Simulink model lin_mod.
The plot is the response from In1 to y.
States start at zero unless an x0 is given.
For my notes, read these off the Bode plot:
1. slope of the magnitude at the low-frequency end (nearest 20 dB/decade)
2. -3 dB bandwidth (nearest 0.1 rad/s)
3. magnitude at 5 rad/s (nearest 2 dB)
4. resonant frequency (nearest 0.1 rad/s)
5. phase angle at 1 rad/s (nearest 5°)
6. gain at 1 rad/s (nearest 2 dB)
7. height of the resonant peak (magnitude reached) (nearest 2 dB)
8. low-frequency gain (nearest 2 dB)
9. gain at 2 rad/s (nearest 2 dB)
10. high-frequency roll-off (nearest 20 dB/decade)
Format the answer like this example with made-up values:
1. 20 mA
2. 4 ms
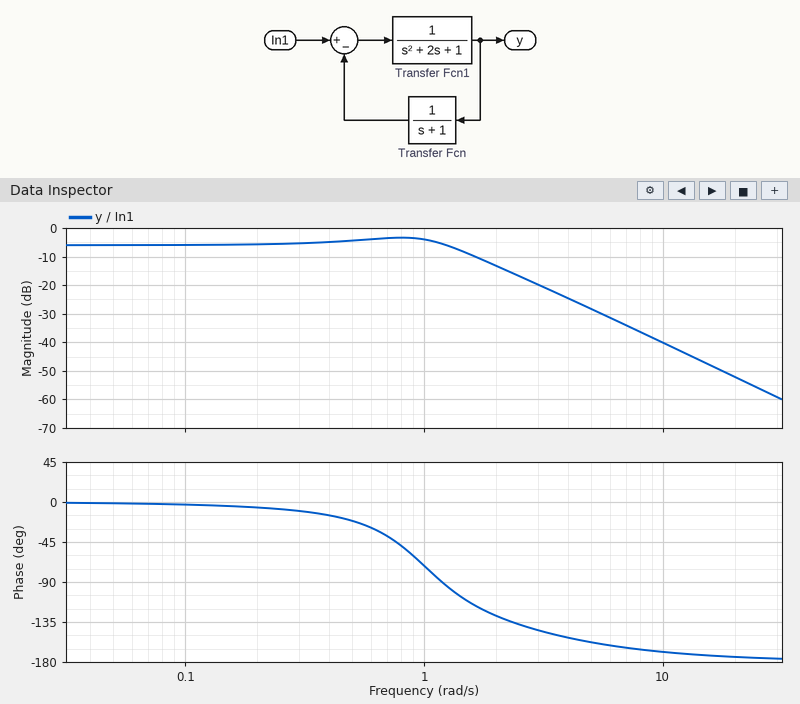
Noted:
1. 0 dB/decade
2. 1.5 rad/s
3. -28 dB
4. 0.8 rad/s
5. -70°
6. -4 dB
7. -4 dB
8. -6 dB
9. -14 dB
10. -40 dB/decade
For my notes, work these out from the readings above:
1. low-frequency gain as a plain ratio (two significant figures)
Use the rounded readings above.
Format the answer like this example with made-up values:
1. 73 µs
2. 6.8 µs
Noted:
1. 0.50
